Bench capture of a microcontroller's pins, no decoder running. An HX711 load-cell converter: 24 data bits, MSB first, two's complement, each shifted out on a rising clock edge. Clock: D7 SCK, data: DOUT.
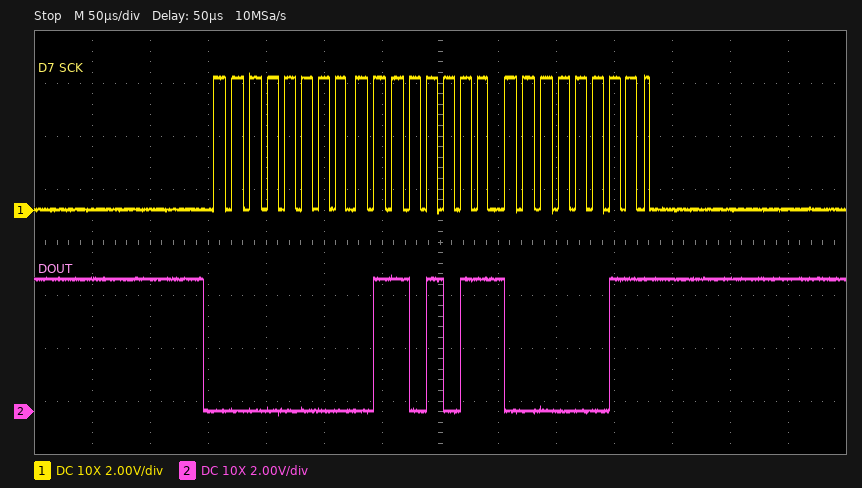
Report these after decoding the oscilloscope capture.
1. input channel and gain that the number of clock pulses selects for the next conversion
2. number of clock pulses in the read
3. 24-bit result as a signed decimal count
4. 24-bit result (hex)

channel A, gain 128
25
27395
0x006B03
